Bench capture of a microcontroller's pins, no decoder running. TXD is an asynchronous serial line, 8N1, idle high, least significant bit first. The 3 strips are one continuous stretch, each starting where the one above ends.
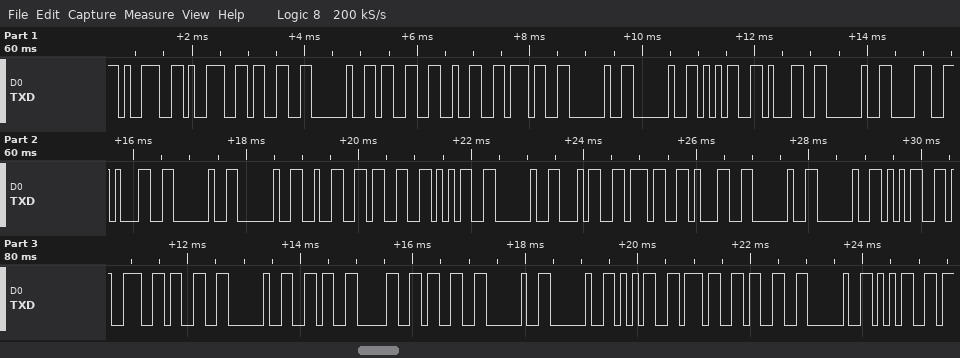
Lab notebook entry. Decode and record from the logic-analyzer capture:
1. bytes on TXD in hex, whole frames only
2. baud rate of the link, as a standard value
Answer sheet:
0x39 0x39 0x33 0x20 0x33 0x32 0x37 0x20 0x20 0x35 0x31 0x20 0x38 0x31 0x20 0x20 0x32 0x33 0x35 0x20 0x34 0x37 0x31 0x20 0x20 0x35 0x39 0x33 0x20 0x36 0x30 0x33 0x20 0x20 0x35 0x37 0x33 0x20 0x35
9600 baud
